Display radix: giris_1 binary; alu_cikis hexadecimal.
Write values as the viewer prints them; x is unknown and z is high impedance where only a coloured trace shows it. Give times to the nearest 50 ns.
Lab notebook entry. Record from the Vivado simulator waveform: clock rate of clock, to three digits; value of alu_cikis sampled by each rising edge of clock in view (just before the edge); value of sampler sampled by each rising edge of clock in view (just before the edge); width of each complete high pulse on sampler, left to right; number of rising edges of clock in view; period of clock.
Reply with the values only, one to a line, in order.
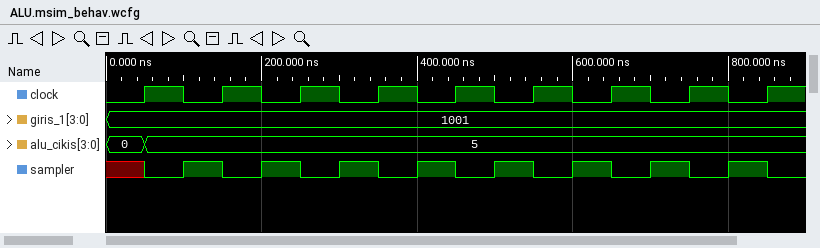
10.0 MHz
0, 5, 5, 5, 5, 5, 5, 5, 5
x 1 1 1 1 1 1 1 1
50 ns, 50 ns, 50 ns, 50 ns, 50 ns, 50 ns, 50 ns, 50 ns
9
100 ns
